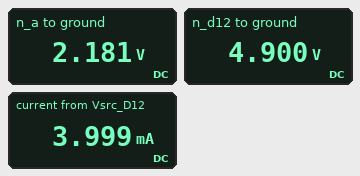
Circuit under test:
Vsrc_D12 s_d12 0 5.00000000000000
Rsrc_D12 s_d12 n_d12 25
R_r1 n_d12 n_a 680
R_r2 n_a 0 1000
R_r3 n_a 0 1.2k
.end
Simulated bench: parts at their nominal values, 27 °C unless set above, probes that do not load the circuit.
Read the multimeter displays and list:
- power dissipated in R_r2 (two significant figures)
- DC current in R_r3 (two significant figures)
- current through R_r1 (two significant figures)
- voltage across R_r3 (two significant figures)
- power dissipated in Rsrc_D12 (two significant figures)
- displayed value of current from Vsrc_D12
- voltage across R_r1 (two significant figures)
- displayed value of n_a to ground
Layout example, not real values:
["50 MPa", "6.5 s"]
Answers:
["4.8 mW", "1.8 mA", "4.0 mA", "2.2 V", "400 µW", "3.999 mA", "2.7 V", "2.181 V"]
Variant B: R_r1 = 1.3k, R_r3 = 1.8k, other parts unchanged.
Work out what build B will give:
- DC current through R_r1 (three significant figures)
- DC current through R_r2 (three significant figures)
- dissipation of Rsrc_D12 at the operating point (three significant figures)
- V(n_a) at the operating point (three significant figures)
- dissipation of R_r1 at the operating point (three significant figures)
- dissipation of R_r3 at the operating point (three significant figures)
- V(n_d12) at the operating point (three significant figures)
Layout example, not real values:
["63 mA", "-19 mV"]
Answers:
["2.54 mA", "1.63 mA", "161 µW", "1.63 V", "8.39 mW", "1.48 mW", "4.94 V"]
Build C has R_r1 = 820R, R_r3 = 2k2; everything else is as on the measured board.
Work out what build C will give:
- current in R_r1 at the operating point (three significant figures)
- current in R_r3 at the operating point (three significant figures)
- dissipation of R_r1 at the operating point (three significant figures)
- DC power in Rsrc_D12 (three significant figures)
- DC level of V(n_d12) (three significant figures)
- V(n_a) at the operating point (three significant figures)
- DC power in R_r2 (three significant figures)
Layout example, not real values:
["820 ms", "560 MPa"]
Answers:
["3.26 mA", "1.02 mA", "8.73 mW", "266 µW", "4.92 V", "2.24 V", "5.03 mW"]
